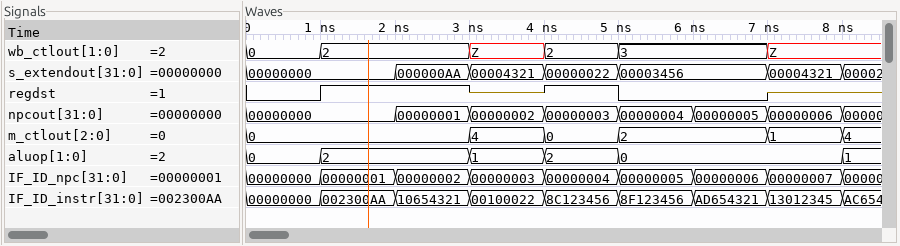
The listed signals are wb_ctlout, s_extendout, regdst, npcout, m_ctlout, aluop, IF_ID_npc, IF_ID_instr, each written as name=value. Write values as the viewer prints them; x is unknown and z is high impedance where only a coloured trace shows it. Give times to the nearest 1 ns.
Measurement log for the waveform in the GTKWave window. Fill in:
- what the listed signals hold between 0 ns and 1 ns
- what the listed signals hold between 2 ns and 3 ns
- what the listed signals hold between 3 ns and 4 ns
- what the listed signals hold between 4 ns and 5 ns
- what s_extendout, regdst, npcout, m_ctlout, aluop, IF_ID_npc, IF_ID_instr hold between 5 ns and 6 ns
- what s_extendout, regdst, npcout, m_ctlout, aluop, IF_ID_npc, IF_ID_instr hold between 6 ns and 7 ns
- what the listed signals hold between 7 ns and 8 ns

wb_ctlout=0, s_extendout=00000000, regdst=0, npcout=00000000, m_ctlout=0, aluop=0, IF_ID_npc=00000000, IF_ID_instr=00000000
wb_ctlout=2, s_extendout=000000AA, regdst=1, npcout=00000001, m_ctlout=0, aluop=2, IF_ID_npc=00000002, IF_ID_instr=10654321
wb_ctlout=Z, s_extendout=00004321, regdst=z, npcout=00000002, m_ctlout=4, aluop=1, IF_ID_npc=00000003, IF_ID_instr=00100022
wb_ctlout=2, s_extendout=00000022, regdst=1, npcout=00000003, m_ctlout=0, aluop=2, IF_ID_npc=00000004, IF_ID_instr=8C123456
s_extendout=00003456, regdst=0, npcout=00000004, m_ctlout=2, aluop=0, IF_ID_npc=00000005, IF_ID_instr=8F123456
s_extendout=00003456, regdst=0, npcout=00000005, m_ctlout=2, aluop=0, IF_ID_npc=00000006, IF_ID_instr=AD654321
wb_ctlout=Z, s_extendout=00004321, regdst=z, npcout=00000006, m_ctlout=1, aluop=0, IF_ID_npc=00000007, IF_ID_instr=13012345
